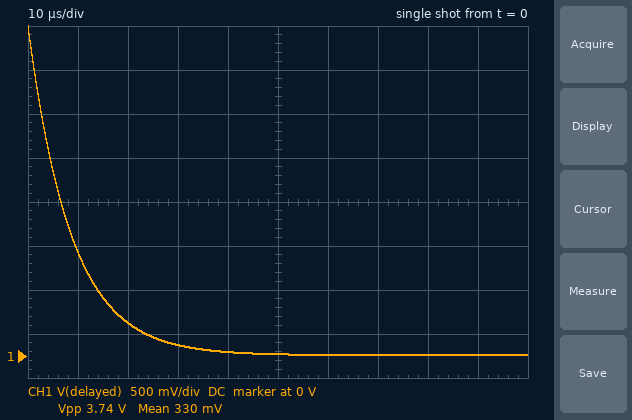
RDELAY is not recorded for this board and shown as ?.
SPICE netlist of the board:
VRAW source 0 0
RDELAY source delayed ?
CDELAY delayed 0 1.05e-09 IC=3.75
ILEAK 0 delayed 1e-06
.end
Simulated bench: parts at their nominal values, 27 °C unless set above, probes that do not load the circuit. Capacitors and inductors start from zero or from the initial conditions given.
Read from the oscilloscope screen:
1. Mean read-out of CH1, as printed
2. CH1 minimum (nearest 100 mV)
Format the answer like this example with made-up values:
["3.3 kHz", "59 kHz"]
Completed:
["330 mV", "0 V"]
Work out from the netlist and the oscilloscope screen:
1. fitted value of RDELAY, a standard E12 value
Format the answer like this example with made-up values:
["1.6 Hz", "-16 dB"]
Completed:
["8.2 kΩ"]
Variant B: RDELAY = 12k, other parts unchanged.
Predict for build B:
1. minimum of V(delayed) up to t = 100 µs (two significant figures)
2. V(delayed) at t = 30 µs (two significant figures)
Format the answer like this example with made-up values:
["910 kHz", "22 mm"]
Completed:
["13 mV", "360 mV"]
